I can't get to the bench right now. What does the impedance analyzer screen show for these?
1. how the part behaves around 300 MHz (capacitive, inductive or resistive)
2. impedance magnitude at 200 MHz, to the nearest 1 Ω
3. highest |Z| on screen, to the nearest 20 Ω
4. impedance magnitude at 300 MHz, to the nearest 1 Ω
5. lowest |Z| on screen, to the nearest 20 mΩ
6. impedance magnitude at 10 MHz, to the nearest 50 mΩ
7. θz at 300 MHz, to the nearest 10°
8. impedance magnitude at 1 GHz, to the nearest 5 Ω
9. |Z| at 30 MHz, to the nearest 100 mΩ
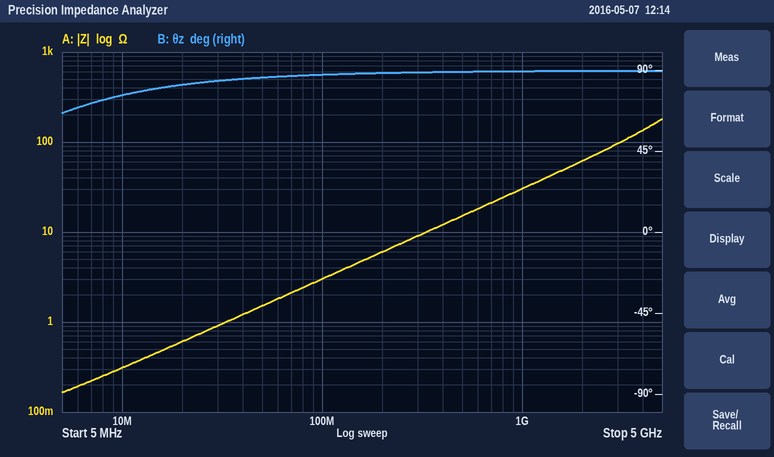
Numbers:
inductive
6 Ω
180 Ω
9 Ω
160 mΩ
300 mΩ
90°
30 Ω
900 mΩ
